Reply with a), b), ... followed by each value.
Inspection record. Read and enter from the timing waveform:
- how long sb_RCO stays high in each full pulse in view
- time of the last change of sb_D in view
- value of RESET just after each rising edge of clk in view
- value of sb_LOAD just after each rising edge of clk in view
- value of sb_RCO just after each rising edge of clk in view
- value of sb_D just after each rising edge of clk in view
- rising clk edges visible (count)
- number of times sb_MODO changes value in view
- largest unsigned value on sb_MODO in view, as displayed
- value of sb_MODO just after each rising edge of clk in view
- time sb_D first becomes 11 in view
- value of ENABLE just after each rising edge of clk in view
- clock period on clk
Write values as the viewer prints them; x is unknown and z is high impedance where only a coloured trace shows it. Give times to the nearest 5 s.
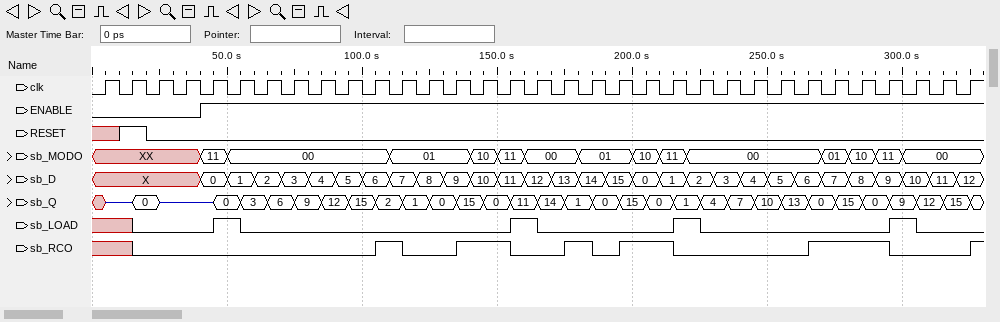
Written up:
a) 10 s, 20 s, 10 s, 20 s, 30 s
b) 320 s
c) x 1 0 0 0 0 0 0 0 0 0 0 0 0 0 0 0 0 0 0 0 0 0 0 0 0 0 0 0 0 0 0 0
d) x 0 0 0 1 0 0 0 0 0 0 0 0 0 0 1 0 0 0 0 0 1 0 0 0 0 0 0 0 1 0 0 0
e) x 0 0 0 0 0 0 0 0 0 1 0 0 1 1 0 0 1 0 1 1 0 0 0 0 0 1 1 1 0 0 0 1
f) X, X, X, X, 0, 1, 2, 3, 4, 5, 6, 7, 8, 9, 10, 11, 12, 13, 14, 15, 0, 1, 2, 3, 4, 5, 6, 7, 8, 9, 10, 11, 12
g) 33
h) 14
i) 11
j) XX, XX, XX, XX, 11, 00, 00, 00, 00, 00, 00, 01, 01, 01, 10, 11, 00, 00, 01, 01, 10, 11, 00, 00, 00, 00, 00, 01, 10, 11, 00, 00, 00
k) 150 s
l) 0 0 0 0 1 1 1 1 1 1 1 1 1 1 1 1 1 1 1 1 1 1 1 1 1 1 1 1 1 1 1 1 1
m) 10 s
